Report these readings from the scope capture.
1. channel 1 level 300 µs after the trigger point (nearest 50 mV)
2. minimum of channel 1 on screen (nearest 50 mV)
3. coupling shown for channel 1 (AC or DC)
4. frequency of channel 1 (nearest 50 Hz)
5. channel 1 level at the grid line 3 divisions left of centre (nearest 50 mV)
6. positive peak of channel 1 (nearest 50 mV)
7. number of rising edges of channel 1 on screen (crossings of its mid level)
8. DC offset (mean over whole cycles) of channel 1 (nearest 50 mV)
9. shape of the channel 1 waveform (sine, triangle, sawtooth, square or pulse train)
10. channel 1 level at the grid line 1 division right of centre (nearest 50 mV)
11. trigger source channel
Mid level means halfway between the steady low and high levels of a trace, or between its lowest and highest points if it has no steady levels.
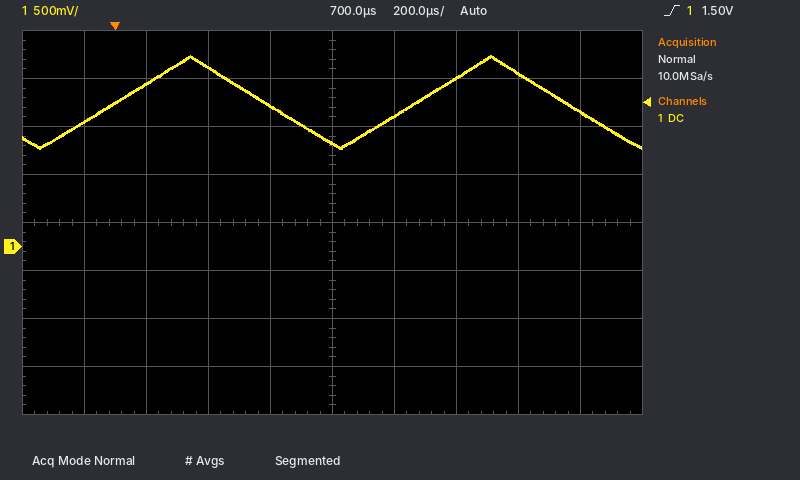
1.85 V
1.00 V
DC
1.05 kHz
1.70 V
2.00 V
2
1.50 V
triangle
1.35 V
channel 1
